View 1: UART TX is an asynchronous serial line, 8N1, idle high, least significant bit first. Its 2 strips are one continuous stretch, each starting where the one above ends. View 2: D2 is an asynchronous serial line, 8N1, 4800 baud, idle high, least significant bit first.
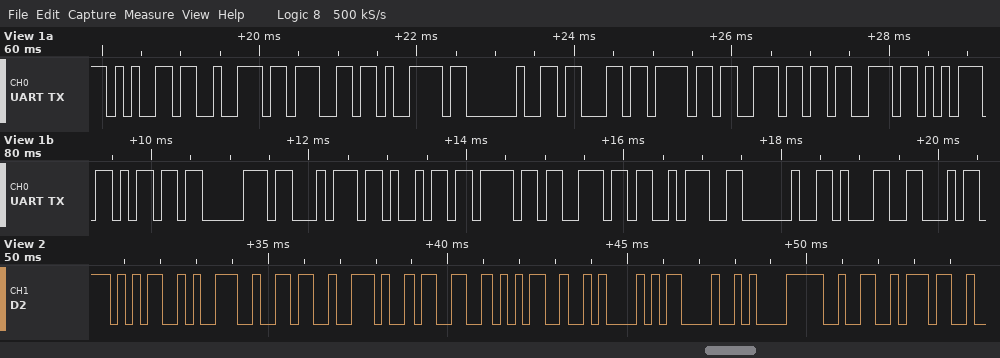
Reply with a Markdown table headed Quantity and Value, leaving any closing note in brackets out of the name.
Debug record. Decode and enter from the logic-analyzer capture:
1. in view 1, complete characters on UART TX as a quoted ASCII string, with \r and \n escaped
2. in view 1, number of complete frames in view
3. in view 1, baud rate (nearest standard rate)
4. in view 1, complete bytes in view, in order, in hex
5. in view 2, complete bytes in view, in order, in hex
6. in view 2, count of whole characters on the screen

| Quantity | Value |
|---|---|
| in view 1, complete characters on UART TX as a quoted ASCII string, with \r and \n escaped | "ergy consumption: 1" |
| in view 1, number of complete frames in view | 19 |
| in view 1, baud rate | 9600 baud |
| in view 1, complete bytes in view, in order, in hex | 65 72 67 79 20 63 6F 6E 73 75 6D 70 74 69 6F 6E 3A 20 31 |
| in view 2, complete bytes in view, in order, in hex | 35 39 36 2E 33 35 0A 0D 0A 32 37 |
| in view 2, count of whole characters on the screen | 11 |
